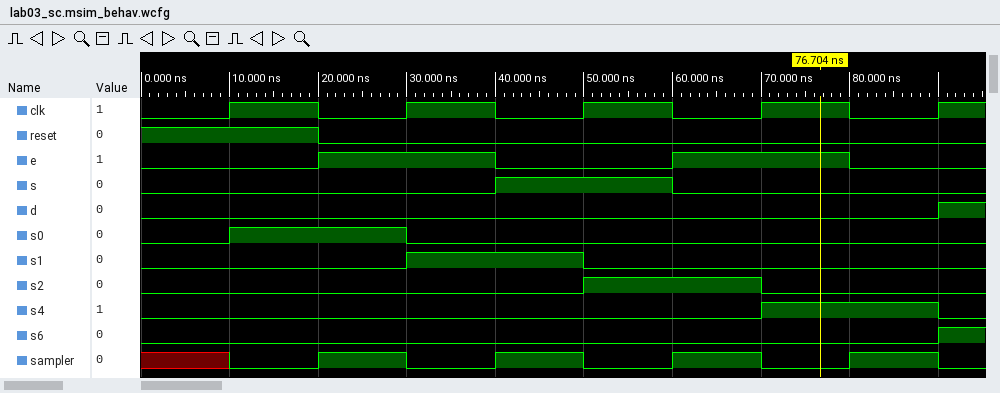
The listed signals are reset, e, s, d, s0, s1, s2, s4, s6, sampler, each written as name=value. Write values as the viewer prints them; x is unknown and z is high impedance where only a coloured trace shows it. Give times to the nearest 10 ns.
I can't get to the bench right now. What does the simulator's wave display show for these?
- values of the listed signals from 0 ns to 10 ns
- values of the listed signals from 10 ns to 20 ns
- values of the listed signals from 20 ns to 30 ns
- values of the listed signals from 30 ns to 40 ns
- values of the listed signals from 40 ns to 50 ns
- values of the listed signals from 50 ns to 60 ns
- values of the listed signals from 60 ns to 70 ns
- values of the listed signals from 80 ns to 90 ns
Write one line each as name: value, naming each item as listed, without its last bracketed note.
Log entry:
values of the listed signals from 0 ns to 10 ns: reset=1, e=0, s=0, d=0, s0=0, s1=0, s2=0, s4=0, s6=0, sampler=x
values of the listed signals from 10 ns to 20 ns: reset=1, e=0, s=0, d=0, s0=1, s1=0, s2=0, s4=0, s6=0, sampler=0
values of the listed signals from 20 ns to 30 ns: reset=0, e=1, s=0, d=0, s0=1, s1=0, s2=0, s4=0, s6=0, sampler=1
values of the listed signals from 30 ns to 40 ns: reset=0, e=1, s=0, d=0, s0=0, s1=1, s2=0, s4=0, s6=0, sampler=0
values of the listed signals from 40 ns to 50 ns: reset=0, e=0, s=1, d=0, s0=0, s1=1, s2=0, s4=0, s6=0, sampler=1
values of the listed signals from 50 ns to 60 ns: reset=0, e=0, s=1, d=0, s0=0, s1=0, s2=1, s4=0, s6=0, sampler=0
values of the listed signals from 60 ns to 70 ns: reset=0, e=1, s=0, d=0, s0=0, s1=0, s2=1, s4=0, s6=0, sampler=1
values of the listed signals from 80 ns to 90 ns: reset=0, e=0, s=0, d=0, s0=0, s1=0, s2=0, s4=1, s6=0, sampler=1
